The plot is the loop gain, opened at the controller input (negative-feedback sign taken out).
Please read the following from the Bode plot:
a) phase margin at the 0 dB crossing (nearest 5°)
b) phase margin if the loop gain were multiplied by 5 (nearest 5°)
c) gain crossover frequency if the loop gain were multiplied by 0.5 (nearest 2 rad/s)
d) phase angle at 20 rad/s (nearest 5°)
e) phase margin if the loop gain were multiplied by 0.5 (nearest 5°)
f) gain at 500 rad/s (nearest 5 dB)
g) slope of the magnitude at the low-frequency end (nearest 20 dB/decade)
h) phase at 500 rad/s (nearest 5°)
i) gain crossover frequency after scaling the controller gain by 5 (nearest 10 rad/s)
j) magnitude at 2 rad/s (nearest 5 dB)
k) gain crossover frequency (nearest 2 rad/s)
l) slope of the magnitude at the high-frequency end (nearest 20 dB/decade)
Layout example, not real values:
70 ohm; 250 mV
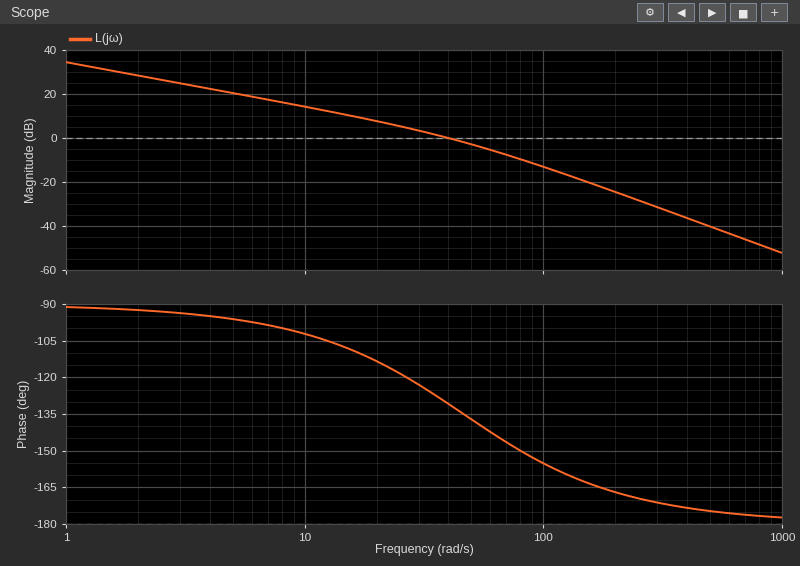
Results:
50°; 25°; 24 rad/s; -115°; 65°; -40 dB; -20 dB/decade; -175°; 110 rad/s; 30 dB; 40 rad/s; -40 dB/decade
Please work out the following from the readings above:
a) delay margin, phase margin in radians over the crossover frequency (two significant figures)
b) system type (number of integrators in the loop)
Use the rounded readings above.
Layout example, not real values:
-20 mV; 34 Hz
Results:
0.022 s; 1
